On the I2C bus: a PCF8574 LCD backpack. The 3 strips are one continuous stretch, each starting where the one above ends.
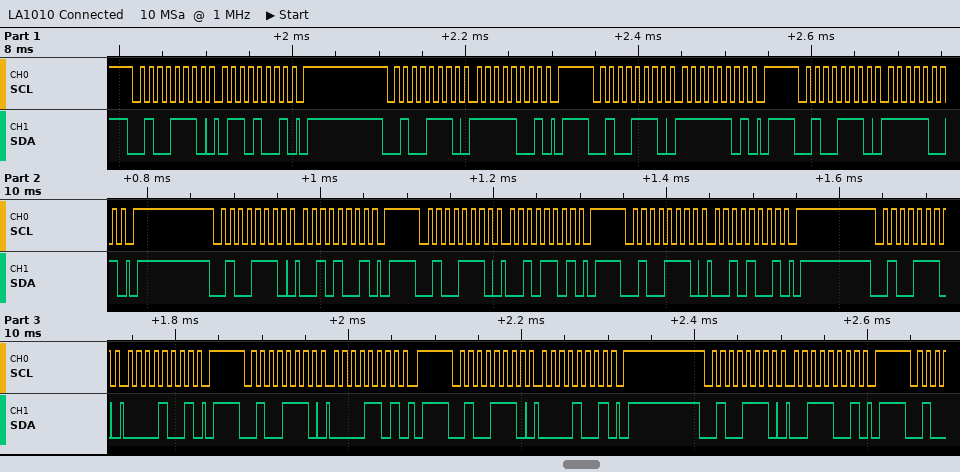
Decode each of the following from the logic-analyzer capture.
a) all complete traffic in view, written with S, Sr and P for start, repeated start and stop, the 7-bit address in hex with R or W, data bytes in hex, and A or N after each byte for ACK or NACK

S 27W A 69 A P S 27W A F9 A P S 27W A FD A P S 27W A F9 A P S 27W A 29 A P S 27W A 2D A P S 27W A 29 A P S 27W A 09 A P S 27W A 0D A P S 27W A 09 A P S 27W A 39 A P
